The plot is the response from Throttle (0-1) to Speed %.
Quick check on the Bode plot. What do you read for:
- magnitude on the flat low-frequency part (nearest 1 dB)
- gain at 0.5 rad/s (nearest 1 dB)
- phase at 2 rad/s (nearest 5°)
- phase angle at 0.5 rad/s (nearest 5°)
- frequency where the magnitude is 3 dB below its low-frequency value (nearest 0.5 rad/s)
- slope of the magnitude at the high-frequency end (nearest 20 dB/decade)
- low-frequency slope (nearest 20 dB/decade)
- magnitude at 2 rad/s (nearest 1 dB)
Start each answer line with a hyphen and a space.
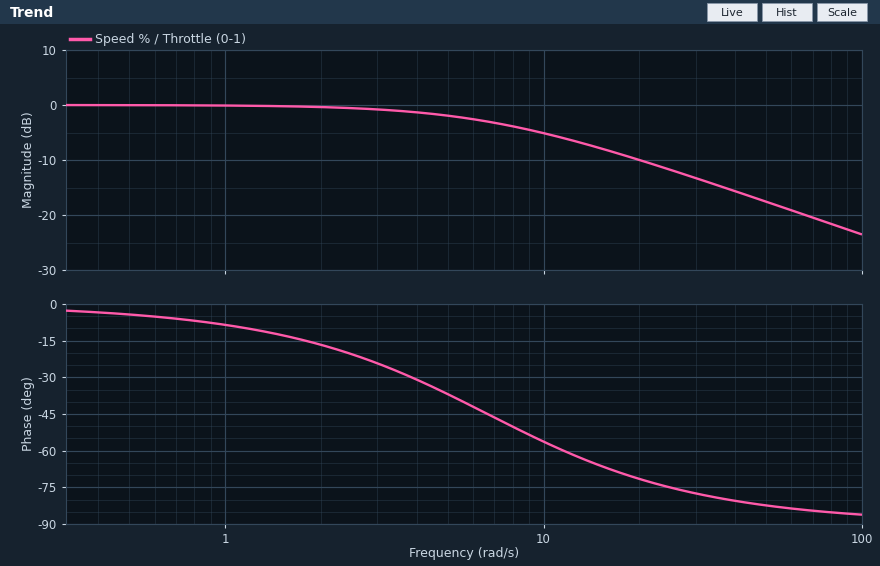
- 0 dB
- 0 dB
- -15°
- -5°
- 6.5 rad/s
- -20 dB/decade
- 0 dB/decade
- 0 dB
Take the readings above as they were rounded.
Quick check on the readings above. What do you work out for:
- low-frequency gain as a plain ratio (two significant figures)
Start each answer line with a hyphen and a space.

- 1.0
